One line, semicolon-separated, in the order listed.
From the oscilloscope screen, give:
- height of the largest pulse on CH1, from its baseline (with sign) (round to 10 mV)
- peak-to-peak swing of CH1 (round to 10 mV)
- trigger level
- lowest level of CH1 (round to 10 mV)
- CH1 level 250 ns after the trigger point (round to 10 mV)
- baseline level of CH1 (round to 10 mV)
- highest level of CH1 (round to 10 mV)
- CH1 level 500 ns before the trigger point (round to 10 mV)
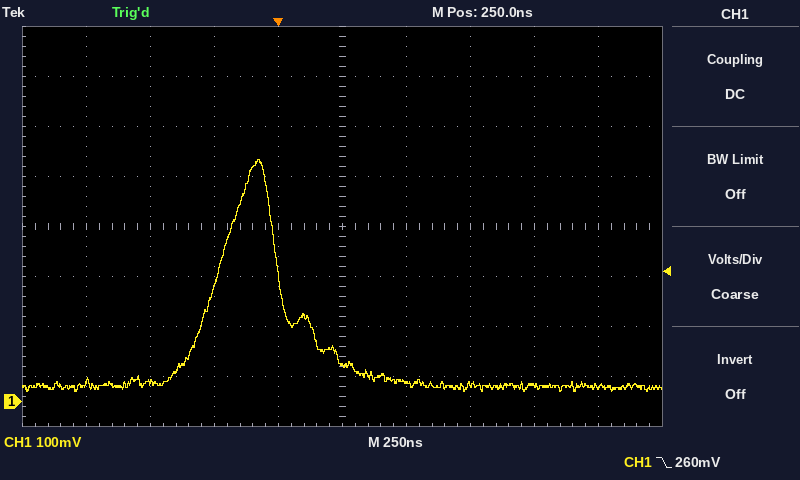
+450 mV; 460 mV; 260 mV; 20 mV; 70 mV; 30 mV; 480 mV; 40 mV
